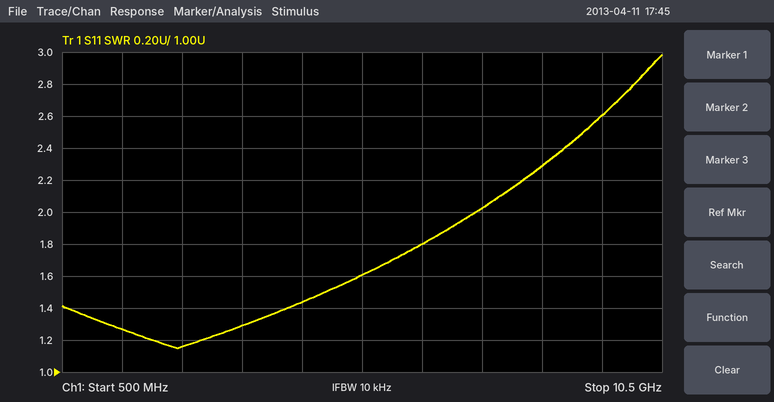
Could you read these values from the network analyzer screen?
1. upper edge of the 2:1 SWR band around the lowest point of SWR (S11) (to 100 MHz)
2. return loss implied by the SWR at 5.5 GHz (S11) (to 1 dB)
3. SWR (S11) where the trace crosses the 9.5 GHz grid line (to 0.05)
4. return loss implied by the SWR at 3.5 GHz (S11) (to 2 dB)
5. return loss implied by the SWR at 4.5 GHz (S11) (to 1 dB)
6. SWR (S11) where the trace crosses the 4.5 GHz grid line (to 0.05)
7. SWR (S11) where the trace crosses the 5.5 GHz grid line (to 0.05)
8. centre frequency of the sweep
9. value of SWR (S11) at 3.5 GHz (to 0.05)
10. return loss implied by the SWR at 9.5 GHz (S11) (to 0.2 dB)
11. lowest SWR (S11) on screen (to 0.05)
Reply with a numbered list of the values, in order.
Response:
1. 7.4 GHz
2. 13 dB
3. 2.60
4. 18 dB
5. 15 dB
6. 1.45
7. 1.60
8. 5.5 GHz
9. 1.30
10. 7.0 dB
11. 1.15
